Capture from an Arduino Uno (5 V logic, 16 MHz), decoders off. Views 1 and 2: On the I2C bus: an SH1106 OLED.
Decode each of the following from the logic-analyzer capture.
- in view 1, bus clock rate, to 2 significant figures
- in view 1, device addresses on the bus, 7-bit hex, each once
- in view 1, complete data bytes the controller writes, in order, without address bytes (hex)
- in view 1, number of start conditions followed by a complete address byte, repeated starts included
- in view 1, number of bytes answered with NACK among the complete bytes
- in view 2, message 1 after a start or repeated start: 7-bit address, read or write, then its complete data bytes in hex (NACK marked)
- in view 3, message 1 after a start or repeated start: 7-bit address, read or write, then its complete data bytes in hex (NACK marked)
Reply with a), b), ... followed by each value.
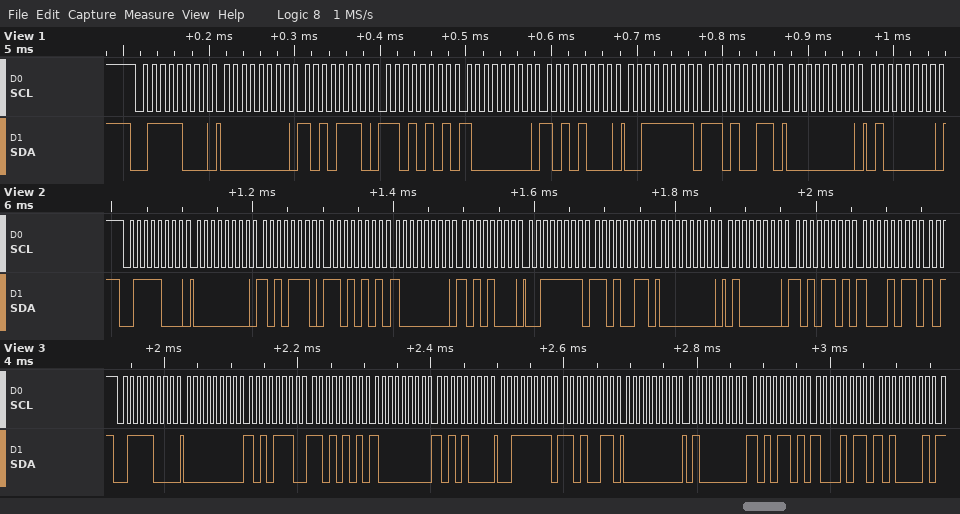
a) 100 kHz
b) 0x3C
c) 00 AE D5 80 A8 3F D3 00 40
d) 1
e) 0
f) 0x3C write: 00 AE D5 80 A8 3F D3 00 40 AD 8B
g) 0x3C write: 00 AE D5 80 A8 3F D3 00 40 AD 8B A1
